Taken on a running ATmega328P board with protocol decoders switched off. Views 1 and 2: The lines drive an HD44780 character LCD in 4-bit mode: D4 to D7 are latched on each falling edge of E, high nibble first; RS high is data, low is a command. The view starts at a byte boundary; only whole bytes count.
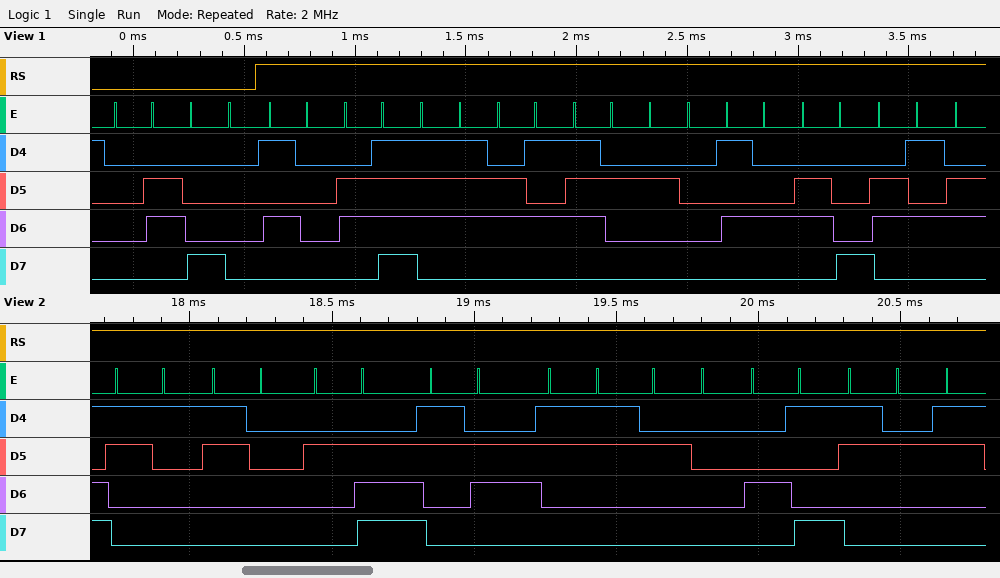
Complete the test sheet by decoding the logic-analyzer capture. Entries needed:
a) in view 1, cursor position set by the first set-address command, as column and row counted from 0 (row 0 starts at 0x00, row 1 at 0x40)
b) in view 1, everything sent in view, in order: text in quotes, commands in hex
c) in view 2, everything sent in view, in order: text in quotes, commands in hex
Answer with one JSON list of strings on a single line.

["column 0, row 0", "0x06 0x80 \"Power The\"", "\"10.63 I2\""]
